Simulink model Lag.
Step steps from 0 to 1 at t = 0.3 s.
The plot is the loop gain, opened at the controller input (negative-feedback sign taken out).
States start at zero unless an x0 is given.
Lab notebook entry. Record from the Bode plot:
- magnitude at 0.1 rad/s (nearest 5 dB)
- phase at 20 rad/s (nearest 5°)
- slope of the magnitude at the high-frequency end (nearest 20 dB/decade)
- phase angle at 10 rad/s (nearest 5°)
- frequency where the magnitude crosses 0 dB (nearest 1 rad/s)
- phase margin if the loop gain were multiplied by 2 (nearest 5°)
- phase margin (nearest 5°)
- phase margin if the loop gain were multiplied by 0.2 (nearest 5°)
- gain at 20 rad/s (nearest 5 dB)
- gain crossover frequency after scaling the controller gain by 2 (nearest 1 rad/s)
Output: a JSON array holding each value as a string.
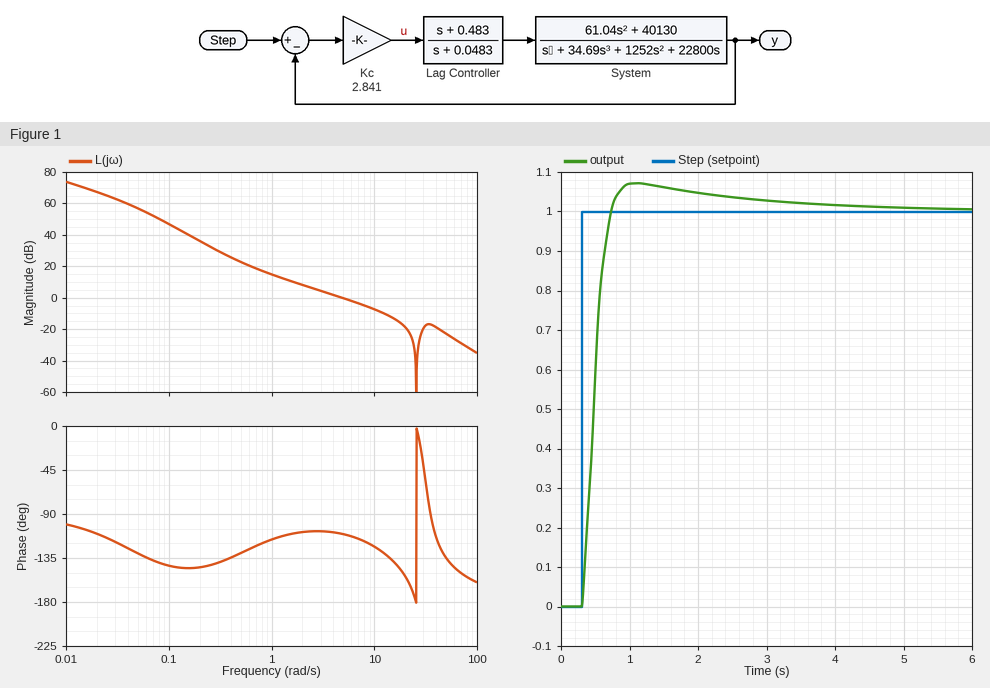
["45 dB", "-155°", "-40 dB/decade", "-125°", "5 rad/s", "60°", "70°", "65°", "-20 dB", "9 rad/s"]
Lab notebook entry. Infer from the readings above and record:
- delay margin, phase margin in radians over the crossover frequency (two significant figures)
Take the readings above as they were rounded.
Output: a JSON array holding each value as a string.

["0.24 s"]
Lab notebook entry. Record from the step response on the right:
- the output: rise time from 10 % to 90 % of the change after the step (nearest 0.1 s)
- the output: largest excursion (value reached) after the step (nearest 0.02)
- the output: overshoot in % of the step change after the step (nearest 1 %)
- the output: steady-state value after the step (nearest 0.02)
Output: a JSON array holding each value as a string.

["0.3 s", "1.08", "7 %", "1.00"]
